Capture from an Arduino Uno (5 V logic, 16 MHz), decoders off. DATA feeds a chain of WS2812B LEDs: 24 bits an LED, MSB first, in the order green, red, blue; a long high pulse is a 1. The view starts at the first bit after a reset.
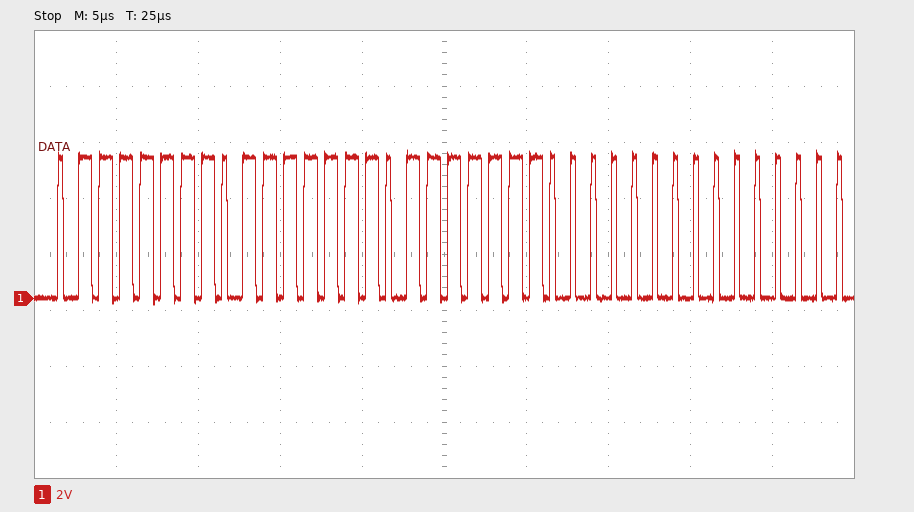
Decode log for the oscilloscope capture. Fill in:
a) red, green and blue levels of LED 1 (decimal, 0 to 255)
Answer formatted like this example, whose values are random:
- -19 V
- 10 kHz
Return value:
- 127, 127, 127
